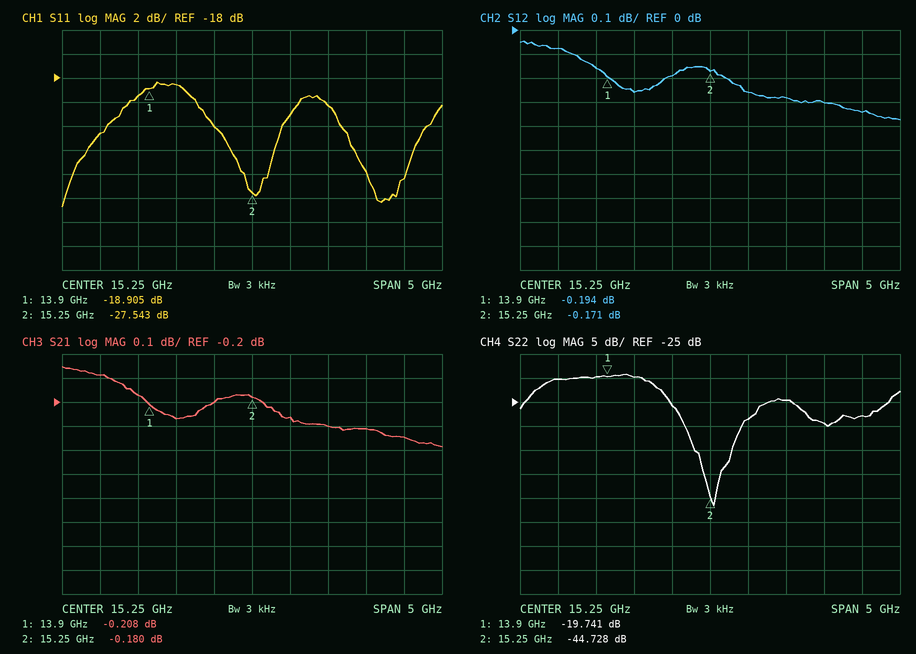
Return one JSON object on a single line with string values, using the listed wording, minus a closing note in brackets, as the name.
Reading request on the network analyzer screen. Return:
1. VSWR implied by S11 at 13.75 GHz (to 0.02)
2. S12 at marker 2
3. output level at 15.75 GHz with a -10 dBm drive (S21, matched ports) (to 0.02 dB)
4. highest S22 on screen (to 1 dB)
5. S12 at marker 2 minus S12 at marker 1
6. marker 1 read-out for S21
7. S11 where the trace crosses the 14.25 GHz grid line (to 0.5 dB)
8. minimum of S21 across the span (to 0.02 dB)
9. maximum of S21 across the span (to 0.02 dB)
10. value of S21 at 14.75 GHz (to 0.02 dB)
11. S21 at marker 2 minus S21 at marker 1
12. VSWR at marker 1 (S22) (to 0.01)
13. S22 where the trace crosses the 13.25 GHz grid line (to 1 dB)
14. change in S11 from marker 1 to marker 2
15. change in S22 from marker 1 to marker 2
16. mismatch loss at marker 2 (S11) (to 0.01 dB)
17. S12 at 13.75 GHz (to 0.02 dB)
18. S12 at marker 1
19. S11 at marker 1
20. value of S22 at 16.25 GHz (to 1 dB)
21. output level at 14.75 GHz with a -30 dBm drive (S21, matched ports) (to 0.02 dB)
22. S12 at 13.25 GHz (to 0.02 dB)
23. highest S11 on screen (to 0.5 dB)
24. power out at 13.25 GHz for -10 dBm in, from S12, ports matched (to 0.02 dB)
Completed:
{"VSWR implied by S11 at 13.75 GHz": "1.24", "S12 at marker 2": "-0.171 dB", "output level at 15.75 GHz with a -10 dBm drive (S21, matched ports)": "-10.26 dBm", "highest S22 on screen": "-19 dB", "S12 at marker 2 minus S12 at marker 1": "0.023 dB", "marker 1 read-out for S21": "-0.208 dB", "S11 where the trace crosses the 14.25 GHz grid line": "-18.5 dB", "minimum of S21 across the span": "-0.38 dB", "maximum of S21 across the span": "-0.06 dB", "value of S21 at 14.75 GHz": "-0.20 dB", "S21 at marker 2 minus S21 at marker 1": "0.028 dB", "VSWR at marker 1 (S22)": "1.23", "S22 where the trace crosses the 13.25 GHz grid line": "-20 dB", "change in S11 from marker 1 to marker 2": "-8.638 dB", "change in S22 from marker 1 to marker 2": "-24.987 dB", "mismatch loss at marker 2 (S11)": "0.01 dB", "S12 at 13.75 GHz": "-0.16 dB", "S12 at marker 1": "-0.194 dB", "S11 at marker 1": "-18.905 dB", "value of S22 at 16.25 GHz": "-25 dB", "output level at 14.75 GHz with a -30 dBm drive (S21, matched ports)": "-30.20 dBm", "S12 at 13.25 GHz": "-0.08 dB", "highest S11 on screen": "-18.5 dB", "power out at 13.25 GHz for -10 dBm in, from S12, ports matched": "-10.08 dBm"}
